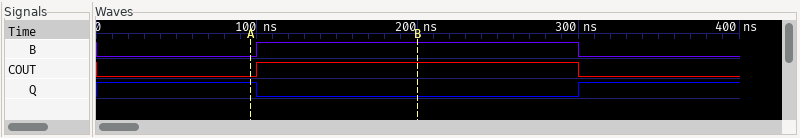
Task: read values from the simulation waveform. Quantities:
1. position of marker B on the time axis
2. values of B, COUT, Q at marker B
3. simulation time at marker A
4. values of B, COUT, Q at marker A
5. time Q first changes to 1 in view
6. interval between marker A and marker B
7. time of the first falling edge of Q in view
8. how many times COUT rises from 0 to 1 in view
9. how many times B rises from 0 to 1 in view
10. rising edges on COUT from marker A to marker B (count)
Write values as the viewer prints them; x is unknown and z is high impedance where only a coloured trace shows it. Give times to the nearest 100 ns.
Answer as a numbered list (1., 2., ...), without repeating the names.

1. 200 ns
2. B=1, COUT=1, Q=0
3. 100 ns
4. B=0, COUT=0, Q=1
5. 300 ns
6. 100 ns
7. 100 ns
8. 1
9. 1
10. 1
